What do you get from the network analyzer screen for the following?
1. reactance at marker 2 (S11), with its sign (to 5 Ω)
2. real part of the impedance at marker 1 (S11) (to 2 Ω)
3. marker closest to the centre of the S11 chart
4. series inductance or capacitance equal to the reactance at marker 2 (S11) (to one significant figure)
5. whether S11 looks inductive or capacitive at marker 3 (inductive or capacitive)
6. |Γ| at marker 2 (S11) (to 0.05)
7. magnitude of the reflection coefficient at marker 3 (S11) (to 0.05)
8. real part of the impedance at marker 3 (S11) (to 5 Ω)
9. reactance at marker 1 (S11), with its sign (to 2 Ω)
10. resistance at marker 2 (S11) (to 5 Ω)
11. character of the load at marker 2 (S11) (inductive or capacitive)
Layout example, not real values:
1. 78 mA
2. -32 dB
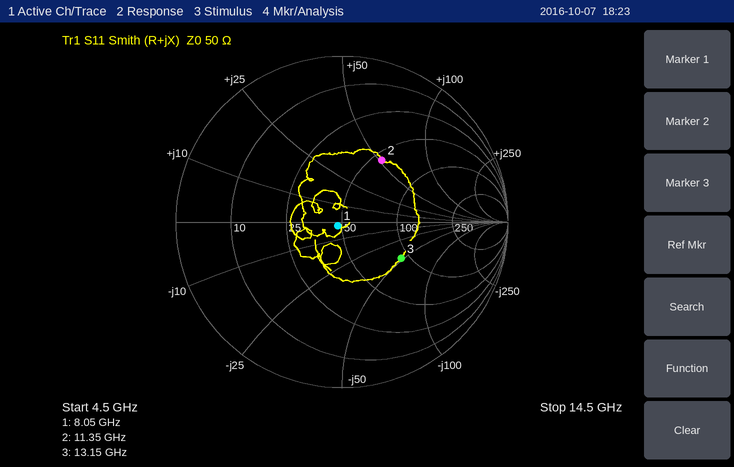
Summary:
1. +50 Ω
2. 48 Ω
3. marker 1
4. 700 pH
5. capacitive
6. 0.45
7. 0.40
8. 90 Ω
9. -2 Ω
10. 55 Ω
11. inductive
